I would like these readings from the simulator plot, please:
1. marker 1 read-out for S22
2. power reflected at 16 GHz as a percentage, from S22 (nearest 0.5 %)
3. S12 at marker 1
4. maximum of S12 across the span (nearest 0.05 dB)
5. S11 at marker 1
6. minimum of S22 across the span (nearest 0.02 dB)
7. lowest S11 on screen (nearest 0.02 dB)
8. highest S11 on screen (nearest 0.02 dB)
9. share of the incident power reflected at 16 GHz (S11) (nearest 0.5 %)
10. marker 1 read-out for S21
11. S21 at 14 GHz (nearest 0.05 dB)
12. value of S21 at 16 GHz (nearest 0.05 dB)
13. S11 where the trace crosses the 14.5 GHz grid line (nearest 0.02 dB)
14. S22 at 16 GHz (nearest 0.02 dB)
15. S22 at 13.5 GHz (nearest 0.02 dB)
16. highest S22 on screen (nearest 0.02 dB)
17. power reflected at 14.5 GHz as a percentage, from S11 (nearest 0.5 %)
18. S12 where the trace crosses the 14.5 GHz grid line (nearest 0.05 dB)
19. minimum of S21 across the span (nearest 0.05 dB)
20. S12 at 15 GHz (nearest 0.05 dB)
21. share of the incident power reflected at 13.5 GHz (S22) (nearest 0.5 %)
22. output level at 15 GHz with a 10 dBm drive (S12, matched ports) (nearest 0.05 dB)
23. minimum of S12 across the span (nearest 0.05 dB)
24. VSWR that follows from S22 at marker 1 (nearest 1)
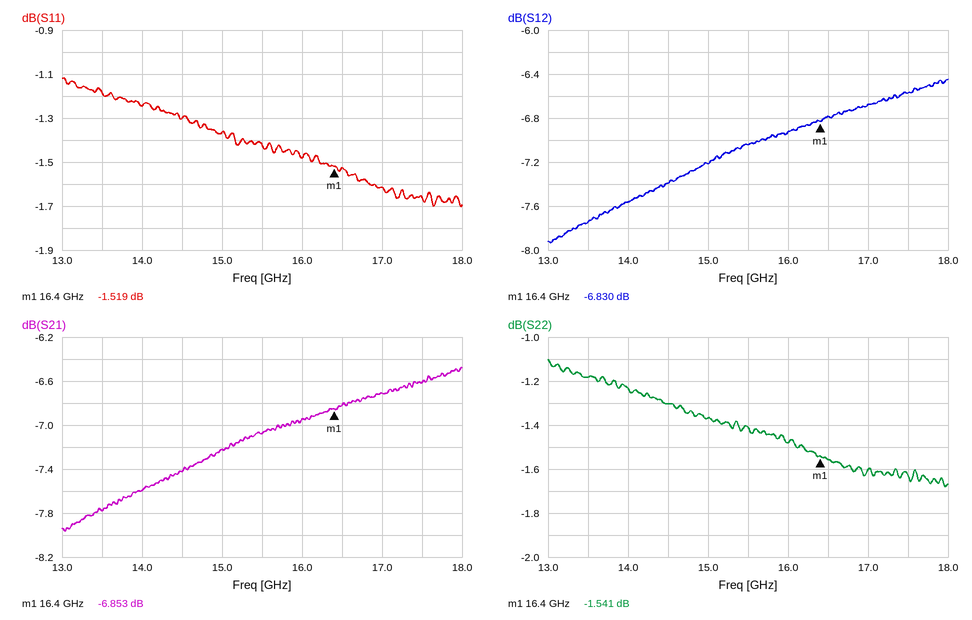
-1.541 dB
71.0 %
-6.830 dB
-6.45 dB
-1.519 dB
-1.68 dB
-1.70 dB
-1.12 dB
71.0 %
-6.853 dB
-7.60 dB
-6.95 dB
-1.30 dB
-1.48 dB
-1.18 dB
-1.10 dB
74.0 %
-7.40 dB
-7.95 dB
-7.20 dB
76.0 %
2.80 dBm
-7.95 dB
11
